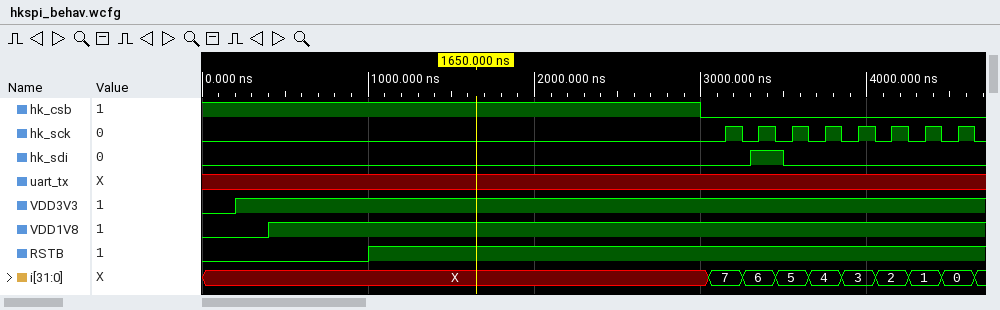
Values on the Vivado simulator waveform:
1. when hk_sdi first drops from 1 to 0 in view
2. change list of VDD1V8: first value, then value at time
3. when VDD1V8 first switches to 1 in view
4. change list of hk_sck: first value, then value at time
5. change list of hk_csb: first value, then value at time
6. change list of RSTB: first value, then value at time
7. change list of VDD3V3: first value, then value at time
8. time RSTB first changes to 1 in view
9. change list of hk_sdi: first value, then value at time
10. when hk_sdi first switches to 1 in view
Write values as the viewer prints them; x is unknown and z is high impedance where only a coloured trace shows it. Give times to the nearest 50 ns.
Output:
3500 ns
0, 1 at 400 ns
400 ns
0, 1 at 3150 ns, 0 at 3250 ns, 1 at 3350 ns, 0 at 3450 ns, 1 at 3550 ns, 0 at 3650 ns, 1 at 3750 ns, 0 at 3850 ns, 1 at 3950 ns, 0 at 4050 ns, 1 at 4150 ns, 0 at 4250 ns, 1 at 4350 ns, 0 at 4450 ns, 1 at 4550 ns, 0 at 4650 ns
1, 0 at 3000 ns
0, 1 at 1000 ns
0, 1 at 200 ns
1000 ns
0, 1 at 3300 ns, 0 at 3500 ns
3300 ns
